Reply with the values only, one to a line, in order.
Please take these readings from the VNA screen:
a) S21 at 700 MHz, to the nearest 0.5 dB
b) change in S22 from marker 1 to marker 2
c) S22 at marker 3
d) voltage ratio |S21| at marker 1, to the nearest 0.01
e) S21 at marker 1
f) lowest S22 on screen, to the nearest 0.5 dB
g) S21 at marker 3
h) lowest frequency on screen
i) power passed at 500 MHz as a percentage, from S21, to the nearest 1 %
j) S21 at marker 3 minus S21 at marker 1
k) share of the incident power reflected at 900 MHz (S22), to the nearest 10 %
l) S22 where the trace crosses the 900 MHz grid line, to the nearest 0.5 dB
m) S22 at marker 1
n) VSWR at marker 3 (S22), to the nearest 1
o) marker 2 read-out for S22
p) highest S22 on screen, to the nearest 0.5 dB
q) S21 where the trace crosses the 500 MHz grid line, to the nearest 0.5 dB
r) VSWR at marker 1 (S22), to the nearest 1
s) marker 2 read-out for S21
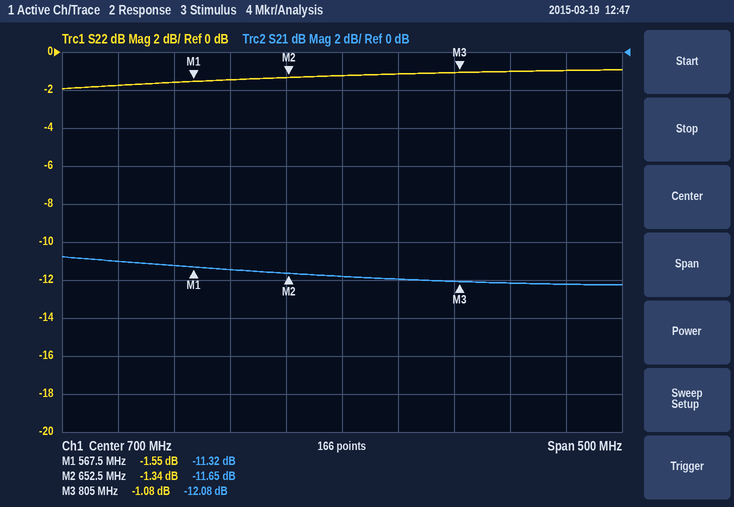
-12.0 dB
0.21 dB
-1.08 dB
0.27
-11.32 dB
-2.0 dB
-12.08 dB
450 MHz
8 %
-0.76 dB
80 %
-1.0 dB
-1.55 dB
16
-1.34 dB
-1.0 dB
-11.0 dB
11
-11.65 dB
